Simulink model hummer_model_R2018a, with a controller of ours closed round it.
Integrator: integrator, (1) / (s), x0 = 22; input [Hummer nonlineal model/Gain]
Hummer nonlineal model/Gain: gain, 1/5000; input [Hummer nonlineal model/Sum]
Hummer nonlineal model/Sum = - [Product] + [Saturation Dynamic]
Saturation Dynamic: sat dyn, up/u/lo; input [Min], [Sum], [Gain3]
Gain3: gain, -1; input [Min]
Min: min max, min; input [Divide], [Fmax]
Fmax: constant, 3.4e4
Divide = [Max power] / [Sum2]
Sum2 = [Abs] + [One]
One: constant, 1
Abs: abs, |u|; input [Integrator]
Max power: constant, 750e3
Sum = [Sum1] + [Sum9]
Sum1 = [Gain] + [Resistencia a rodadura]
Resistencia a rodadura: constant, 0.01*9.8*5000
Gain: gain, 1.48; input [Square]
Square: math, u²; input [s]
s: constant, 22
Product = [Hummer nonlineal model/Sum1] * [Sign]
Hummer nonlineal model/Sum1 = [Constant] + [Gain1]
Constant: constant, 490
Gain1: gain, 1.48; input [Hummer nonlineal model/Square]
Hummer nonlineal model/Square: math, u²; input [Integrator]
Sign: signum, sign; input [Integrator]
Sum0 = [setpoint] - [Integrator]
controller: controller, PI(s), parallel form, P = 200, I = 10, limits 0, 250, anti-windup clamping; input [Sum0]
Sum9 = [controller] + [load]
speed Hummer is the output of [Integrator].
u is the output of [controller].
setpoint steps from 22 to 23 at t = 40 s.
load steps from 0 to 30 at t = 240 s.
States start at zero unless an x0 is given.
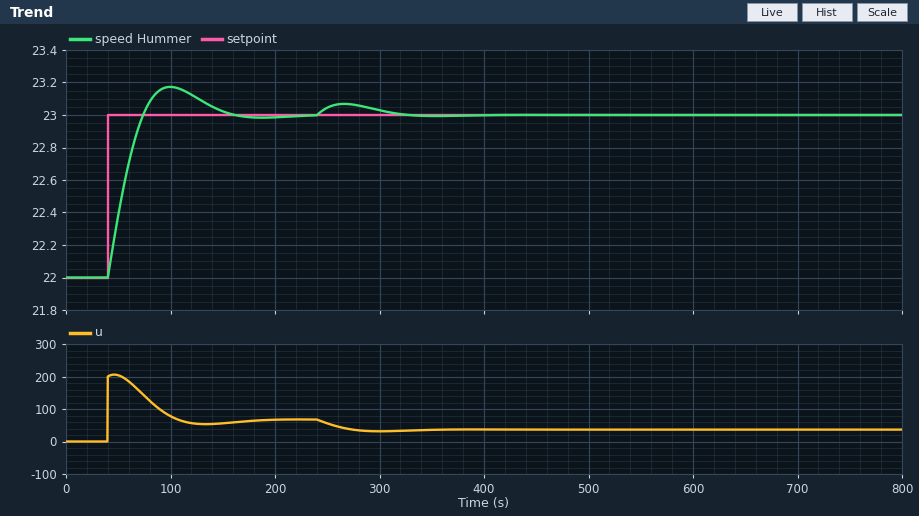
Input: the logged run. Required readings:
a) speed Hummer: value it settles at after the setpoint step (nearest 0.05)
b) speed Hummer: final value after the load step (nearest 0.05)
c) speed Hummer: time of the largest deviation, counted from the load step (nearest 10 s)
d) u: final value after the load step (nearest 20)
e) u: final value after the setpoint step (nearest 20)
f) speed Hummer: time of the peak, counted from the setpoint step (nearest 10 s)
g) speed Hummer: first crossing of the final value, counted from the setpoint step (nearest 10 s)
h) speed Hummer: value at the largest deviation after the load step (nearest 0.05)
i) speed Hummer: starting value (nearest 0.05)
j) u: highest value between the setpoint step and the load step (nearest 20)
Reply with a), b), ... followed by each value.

a) 23.00
b) 23.00
c) 30 s
d) 40
e) 60
f) 60 s
g) 30 s
h) 23.05
i) 22.00
j) 200
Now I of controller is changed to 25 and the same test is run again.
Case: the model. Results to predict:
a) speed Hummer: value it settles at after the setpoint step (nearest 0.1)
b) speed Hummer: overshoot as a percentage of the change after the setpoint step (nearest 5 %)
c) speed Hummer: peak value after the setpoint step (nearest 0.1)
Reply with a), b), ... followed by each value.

a) 23.0
b) 25 %
c) 23.3
